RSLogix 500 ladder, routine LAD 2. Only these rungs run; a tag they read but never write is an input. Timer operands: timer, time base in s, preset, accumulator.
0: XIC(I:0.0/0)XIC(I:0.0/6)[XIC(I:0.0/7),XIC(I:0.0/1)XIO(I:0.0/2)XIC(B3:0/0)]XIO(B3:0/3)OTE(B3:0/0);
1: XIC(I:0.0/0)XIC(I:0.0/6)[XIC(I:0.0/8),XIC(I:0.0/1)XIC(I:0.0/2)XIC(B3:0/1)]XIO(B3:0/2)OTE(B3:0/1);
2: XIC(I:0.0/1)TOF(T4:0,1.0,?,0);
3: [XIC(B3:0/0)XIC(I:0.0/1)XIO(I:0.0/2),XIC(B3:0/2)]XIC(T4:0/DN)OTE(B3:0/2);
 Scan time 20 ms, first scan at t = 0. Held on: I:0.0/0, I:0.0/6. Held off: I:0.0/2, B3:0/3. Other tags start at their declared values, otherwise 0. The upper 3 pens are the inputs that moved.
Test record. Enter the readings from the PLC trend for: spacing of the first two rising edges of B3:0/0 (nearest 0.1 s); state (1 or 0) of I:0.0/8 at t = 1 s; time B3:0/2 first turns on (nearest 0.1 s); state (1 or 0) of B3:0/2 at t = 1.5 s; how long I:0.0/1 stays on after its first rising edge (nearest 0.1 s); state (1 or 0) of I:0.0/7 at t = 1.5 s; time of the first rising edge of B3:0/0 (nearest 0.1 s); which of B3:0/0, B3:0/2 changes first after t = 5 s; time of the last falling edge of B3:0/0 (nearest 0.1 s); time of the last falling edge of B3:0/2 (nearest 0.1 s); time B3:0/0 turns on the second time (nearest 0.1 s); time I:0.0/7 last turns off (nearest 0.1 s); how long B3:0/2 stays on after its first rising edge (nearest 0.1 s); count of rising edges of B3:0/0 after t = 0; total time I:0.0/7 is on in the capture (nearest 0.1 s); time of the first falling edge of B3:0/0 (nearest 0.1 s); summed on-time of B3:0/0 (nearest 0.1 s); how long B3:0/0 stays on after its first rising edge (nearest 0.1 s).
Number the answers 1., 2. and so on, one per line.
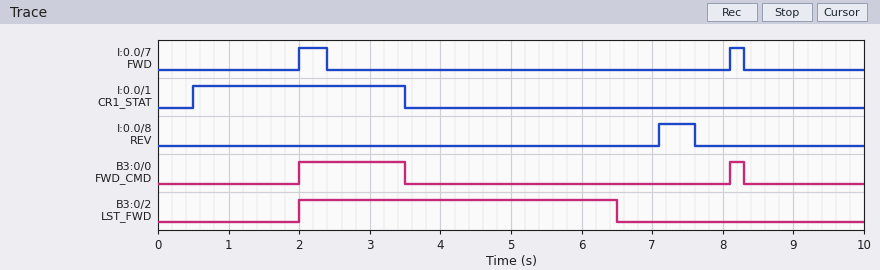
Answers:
1. 6.1 s
2. 0
3. 2.0 s
4. 0
5. 3.0 s
6. 0
7. 2.0 s
8. B3:0/2
9. 8.3 s
10. 6.5 s
11. 8.1 s
12. 8.3 s
13. 4.5 s
14. 2
15. 0.6 s
16. 3.5 s
17. 1.7 s
18. 1.5 s
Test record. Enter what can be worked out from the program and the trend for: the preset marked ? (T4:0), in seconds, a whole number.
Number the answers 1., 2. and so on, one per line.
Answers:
1. 3 s
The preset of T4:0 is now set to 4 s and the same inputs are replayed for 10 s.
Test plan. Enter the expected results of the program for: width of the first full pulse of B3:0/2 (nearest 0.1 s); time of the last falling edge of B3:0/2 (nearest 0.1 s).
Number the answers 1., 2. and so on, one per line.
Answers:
1. 5.5 s
2. 7.5 s
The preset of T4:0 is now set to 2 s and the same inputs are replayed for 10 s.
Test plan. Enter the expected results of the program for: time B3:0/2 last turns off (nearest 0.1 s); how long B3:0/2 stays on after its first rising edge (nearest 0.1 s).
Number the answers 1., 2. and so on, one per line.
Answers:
1. 5.5 s
2. 3.5 s
